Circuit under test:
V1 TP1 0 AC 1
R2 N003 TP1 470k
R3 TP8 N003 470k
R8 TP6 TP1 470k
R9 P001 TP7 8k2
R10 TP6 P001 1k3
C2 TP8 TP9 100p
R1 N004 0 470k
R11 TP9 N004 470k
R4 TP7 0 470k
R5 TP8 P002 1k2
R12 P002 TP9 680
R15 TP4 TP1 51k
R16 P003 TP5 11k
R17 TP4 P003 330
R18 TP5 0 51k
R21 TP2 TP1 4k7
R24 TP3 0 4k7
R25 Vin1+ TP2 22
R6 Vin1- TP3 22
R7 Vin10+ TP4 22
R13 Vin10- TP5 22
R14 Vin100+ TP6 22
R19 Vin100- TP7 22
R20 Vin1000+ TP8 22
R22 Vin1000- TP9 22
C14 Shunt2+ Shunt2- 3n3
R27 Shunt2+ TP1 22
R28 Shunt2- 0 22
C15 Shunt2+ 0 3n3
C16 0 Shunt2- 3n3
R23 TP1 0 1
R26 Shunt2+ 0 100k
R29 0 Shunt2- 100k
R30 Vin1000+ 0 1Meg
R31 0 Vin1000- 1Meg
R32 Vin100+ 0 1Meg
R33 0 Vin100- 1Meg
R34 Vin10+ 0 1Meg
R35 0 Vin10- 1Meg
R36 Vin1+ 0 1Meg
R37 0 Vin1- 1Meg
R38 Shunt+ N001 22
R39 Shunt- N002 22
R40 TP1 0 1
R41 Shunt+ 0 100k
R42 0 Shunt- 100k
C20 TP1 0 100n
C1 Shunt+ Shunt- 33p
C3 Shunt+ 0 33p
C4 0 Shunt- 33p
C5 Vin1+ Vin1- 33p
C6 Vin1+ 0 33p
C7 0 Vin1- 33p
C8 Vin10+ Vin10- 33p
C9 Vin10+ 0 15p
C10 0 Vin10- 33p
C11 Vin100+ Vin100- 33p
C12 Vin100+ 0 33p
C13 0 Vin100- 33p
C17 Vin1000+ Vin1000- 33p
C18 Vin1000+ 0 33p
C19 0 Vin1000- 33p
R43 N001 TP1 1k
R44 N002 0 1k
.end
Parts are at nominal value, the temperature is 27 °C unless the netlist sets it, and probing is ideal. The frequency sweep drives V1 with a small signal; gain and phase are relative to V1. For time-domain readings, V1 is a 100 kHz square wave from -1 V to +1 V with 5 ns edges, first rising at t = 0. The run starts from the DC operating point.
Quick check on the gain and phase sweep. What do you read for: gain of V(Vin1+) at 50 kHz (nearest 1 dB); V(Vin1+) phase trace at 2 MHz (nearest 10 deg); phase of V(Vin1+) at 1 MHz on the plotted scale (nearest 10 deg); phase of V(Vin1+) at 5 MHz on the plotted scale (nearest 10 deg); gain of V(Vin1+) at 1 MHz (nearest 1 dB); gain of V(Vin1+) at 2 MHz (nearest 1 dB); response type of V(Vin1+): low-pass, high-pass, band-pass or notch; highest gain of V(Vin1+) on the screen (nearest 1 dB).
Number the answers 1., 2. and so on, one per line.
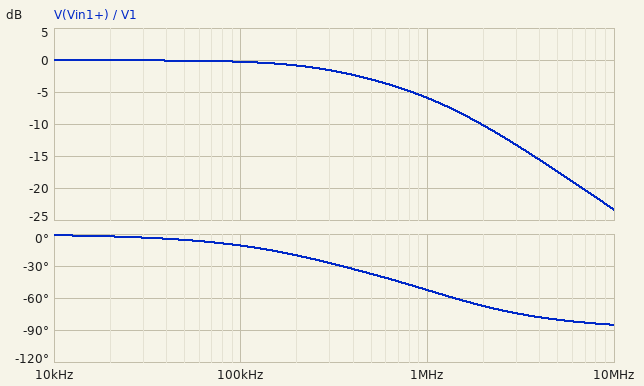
1. 0 dB
2. -70 deg
3. -50 deg
4. -80 deg
5. -6 dB
6. -10 dB
7. low-pass
8. 0 dB
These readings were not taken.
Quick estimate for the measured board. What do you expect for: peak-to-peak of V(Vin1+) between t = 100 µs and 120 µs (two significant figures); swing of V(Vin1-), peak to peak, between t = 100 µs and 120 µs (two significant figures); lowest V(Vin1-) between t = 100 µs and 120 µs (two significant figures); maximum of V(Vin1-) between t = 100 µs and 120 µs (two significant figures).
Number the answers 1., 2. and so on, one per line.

1. 2.0 V
2. 770 mV
3. -380 mV
4. 380 mV
